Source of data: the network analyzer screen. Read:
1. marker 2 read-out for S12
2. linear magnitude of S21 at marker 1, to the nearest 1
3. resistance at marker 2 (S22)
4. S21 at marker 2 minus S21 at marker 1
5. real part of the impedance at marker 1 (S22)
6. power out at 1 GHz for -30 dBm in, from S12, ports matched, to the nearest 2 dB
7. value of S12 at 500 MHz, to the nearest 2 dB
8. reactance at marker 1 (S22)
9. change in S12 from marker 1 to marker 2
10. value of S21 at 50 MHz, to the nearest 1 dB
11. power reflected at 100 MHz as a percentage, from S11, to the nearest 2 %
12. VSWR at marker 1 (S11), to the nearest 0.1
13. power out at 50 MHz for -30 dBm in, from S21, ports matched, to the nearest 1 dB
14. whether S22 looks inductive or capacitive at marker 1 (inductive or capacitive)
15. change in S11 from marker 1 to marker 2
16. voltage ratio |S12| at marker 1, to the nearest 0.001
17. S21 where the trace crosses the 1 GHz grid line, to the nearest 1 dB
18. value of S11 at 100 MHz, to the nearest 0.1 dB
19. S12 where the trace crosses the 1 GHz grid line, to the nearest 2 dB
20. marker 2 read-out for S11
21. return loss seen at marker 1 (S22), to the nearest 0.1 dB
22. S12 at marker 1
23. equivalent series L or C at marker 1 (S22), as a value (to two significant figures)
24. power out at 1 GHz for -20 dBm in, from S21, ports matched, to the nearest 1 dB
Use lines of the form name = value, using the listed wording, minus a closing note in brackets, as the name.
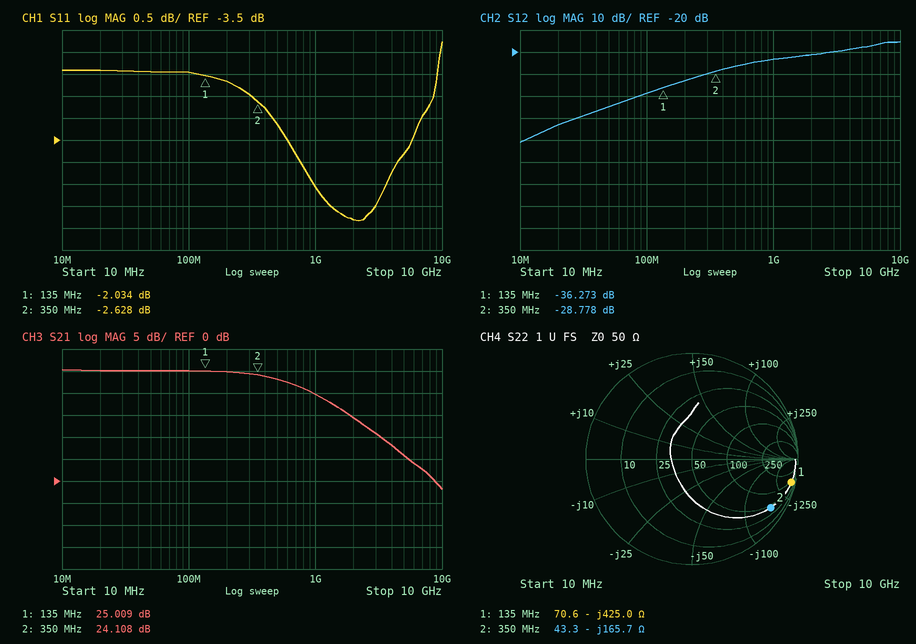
marker 2 read-out for S12 = -28.778 dB
linear magnitude of S21 at marker 1, to the nearest 1 = 18
resistance at marker 2 = 43.3 Ω
S21 at marker 2 minus S21 at marker 1 = -0.901 dB
real part of the impedance at marker 1 = 70.6 Ω
power out at 1 GHz for -30 dBm in, from S12, ports matched, to the nearest 2 dB = -54 dBm
value of S12 at 500 MHz, to the nearest 2 dB = -26 dB
reactance at marker 1 = -425.0 Ω
change in S12 from marker 1 to marker 2 = 7.495 dB
value of S21 at 50 MHz, to the nearest 1 dB = 25 dB
power reflected at 100 MHz as a percentage, from S11, to the nearest 2 % = 64 %
VSWR at marker 1 (S11), to the nearest 0.1 = 8.6
power out at 50 MHz for -30 dBm in, from S21, ports matched, to the nearest 1 dB = -5 dBm
whether S22 looks inductive or capacitive at marker 1 = capacitive
change in S11 from marker 1 to marker 2 = -0.594 dB
voltage ratio |S12| at marker 1, to the nearest 0.001 = 0.015
S21 where the trace crosses the 1 GHz grid line, to the nearest 1 dB = 20 dB
value of S11 at 100 MHz, to the nearest 0.1 dB = -2.0 dB
S12 where the trace crosses the 1 GHz grid line, to the nearest 2 dB = -24 dB
marker 2 read-out for S11 = -2.628 dB
return loss seen at marker 1 (S22), to the nearest 0.1 dB = 0.3 dB
S12 at marker 1 = -36.273 dB
equivalent series L or C at marker 1 (S22), as a value = 2.8 pF
power out at 1 GHz for -20 dBm in, from S21, ports matched, to the nearest 1 dB = 0 dBm
